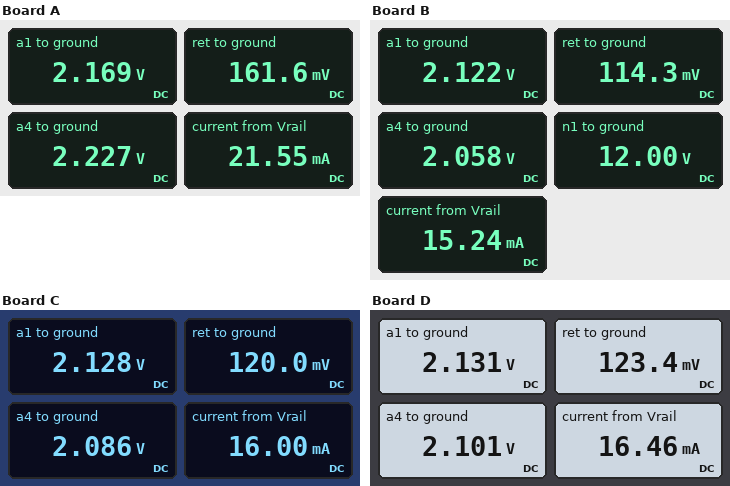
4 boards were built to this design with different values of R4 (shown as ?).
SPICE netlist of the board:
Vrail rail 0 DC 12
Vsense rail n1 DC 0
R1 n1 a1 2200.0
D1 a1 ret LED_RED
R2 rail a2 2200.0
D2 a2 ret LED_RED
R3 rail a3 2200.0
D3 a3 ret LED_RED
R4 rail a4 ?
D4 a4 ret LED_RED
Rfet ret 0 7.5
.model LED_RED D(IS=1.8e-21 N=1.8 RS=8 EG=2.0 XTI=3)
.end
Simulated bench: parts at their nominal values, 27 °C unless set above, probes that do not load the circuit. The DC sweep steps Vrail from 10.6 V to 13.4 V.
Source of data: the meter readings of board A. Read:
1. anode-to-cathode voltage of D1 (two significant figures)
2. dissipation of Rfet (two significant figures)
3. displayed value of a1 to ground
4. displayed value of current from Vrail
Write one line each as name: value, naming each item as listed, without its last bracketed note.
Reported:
anode-to-cathode voltage of D1: 2.0 V
dissipation of Rfet: 3.5 mW
displayed value of a1 to ground: 2.169 V
displayed value of current from Vrail: 21.55 mA
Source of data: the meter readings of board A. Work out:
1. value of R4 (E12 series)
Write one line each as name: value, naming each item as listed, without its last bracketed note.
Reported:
value of R4: 1.2 kΩ
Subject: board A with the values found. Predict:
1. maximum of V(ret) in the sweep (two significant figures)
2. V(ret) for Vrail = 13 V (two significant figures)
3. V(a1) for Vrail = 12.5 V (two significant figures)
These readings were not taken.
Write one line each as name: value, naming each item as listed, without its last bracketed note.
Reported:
maximum of V(ret) in the sweep: 180 mV
V(ret) for Vrail = 13 V: 180 mV
V(a1) for Vrail = 12.5 V: 2.2 V
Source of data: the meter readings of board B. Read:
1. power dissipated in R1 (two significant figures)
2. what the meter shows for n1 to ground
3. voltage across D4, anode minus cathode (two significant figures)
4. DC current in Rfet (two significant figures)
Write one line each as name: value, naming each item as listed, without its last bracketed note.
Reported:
power dissipated in R1: 44 mW
what the meter shows for n1 to ground: 12.00 V
voltage across D4, anode minus cathode: 1.9 V
DC current in Rfet: 15 mA
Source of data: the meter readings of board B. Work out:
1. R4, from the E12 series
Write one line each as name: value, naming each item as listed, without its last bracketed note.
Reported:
R4, from the E12 series: 5.6 kΩ
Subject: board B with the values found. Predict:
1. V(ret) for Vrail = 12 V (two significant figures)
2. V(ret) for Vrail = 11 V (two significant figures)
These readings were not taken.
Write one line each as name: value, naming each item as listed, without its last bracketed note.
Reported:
V(ret) for Vrail = 12 V: 110 mV
V(ret) for Vrail = 11 V: 100 mV
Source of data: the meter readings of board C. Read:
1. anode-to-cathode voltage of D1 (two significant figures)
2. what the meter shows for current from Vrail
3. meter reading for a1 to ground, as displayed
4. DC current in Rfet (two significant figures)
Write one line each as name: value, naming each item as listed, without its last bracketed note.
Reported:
anode-to-cathode voltage of D1: 2.0 V
what the meter shows for current from Vrail: 16.00 mA
meter reading for a1 to ground, as displayed: 2.128 V
DC current in Rfet: 16 mA
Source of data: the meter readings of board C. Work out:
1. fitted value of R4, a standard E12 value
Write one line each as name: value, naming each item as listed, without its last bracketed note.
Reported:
fitted value of R4, a standard E12 value: 3.9 kΩ
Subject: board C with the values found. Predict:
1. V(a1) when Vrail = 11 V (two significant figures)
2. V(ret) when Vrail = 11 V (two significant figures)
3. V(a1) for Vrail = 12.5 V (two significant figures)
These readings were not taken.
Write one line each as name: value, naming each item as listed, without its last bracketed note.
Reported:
V(a1) when Vrail = 11 V: 2.1 V
V(ret) when Vrail = 11 V: 110 mV
V(a1) for Vrail = 12.5 V: 2.1 V
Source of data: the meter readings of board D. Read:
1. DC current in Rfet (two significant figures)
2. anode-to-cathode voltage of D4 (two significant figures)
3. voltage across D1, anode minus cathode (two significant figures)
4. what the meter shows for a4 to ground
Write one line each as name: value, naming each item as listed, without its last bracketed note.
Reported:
DC current in Rfet: 16 mA
anode-to-cathode voltage of D4: 2.0 V
voltage across D1, anode minus cathode: 2.0 V
what the meter shows for a4 to ground: 2.101 V
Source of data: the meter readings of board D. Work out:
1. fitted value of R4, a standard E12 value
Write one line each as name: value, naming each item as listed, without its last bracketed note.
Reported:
fitted value of R4, a standard E12 value: 3.3 kΩ
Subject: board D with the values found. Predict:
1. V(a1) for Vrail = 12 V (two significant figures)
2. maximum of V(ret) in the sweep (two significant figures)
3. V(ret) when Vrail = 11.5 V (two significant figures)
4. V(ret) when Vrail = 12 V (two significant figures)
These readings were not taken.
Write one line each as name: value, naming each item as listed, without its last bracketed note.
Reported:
V(a1) for Vrail = 12 V: 2.1 V
maximum of V(ret) in the sweep: 140 mV
V(ret) when Vrail = 11.5 V: 120 mV
V(ret) when Vrail = 12 V: 120 mV
